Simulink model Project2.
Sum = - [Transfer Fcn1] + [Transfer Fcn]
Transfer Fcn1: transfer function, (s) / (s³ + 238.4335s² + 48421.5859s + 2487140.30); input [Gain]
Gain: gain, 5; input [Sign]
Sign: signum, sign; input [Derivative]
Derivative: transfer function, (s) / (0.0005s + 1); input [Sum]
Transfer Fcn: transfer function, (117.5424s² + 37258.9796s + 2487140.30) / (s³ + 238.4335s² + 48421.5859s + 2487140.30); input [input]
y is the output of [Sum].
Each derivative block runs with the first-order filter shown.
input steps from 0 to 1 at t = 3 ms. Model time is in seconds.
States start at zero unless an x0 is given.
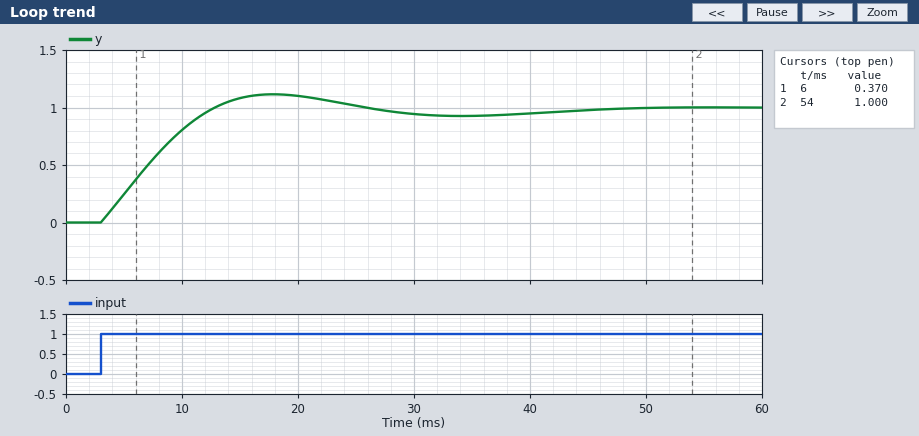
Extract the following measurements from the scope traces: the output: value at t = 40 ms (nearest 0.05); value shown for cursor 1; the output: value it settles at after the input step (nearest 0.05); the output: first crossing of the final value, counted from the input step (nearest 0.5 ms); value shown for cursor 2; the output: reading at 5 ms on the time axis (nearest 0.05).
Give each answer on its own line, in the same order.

0.95
0.370
1.00
10.0 ms
1.000
0.25
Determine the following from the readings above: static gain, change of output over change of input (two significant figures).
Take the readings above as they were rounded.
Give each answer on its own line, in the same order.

1.0
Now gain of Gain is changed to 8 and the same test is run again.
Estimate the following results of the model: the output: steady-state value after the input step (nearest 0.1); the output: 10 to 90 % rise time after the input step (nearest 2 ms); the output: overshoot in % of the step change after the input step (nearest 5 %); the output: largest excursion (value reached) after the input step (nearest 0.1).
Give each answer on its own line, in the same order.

1.0
8 ms
10 %
1.1
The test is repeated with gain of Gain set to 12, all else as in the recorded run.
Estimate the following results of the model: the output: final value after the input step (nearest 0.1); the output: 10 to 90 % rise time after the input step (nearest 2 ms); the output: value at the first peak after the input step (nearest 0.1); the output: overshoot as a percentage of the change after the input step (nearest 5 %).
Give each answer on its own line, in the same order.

1.0
8 ms
1.1
10 %
